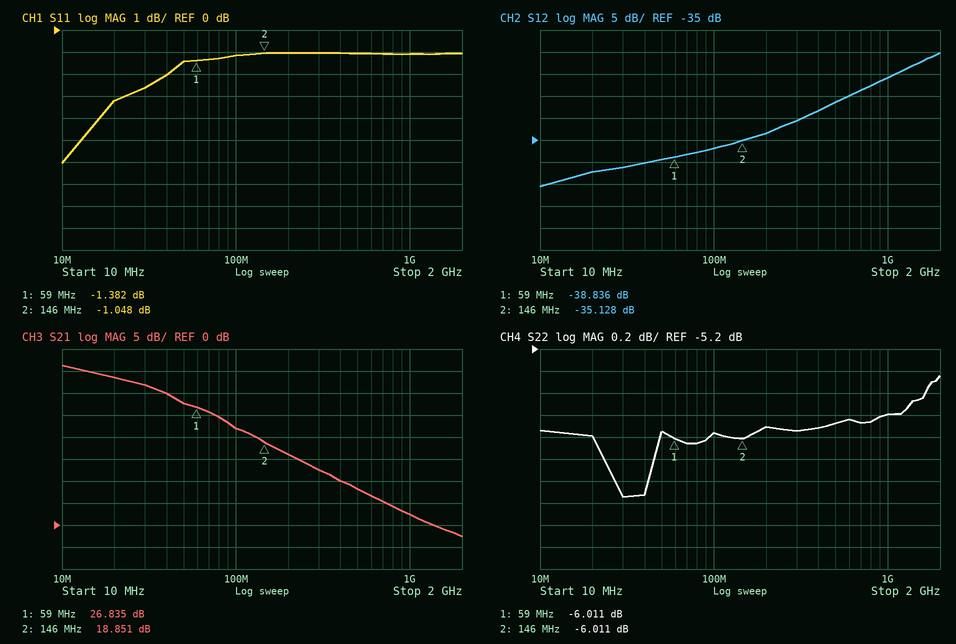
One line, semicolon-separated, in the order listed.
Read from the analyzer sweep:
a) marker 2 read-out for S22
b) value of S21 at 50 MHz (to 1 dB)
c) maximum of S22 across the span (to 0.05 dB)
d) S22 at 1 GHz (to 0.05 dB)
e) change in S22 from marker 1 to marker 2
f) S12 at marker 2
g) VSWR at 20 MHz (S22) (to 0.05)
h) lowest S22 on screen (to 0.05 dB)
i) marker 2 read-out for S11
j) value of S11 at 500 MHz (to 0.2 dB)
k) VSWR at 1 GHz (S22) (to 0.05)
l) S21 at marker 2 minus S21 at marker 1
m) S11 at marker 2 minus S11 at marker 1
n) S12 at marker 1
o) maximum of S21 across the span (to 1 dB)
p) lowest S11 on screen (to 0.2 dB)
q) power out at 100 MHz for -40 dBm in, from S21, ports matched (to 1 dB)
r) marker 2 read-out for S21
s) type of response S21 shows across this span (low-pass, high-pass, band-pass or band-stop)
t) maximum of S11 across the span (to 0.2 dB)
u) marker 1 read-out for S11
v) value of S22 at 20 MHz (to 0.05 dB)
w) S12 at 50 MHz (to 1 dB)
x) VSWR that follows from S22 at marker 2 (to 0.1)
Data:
-6.011 dB; 28 dB; -5.45 dB; -5.80 dB; 0.000 dB; -35.128 dB; 3.00; -6.55 dB; -1.048 dB; -1.0 dB; 3.10; -7.984 dB; 0.334 dB; -38.836 dB; 36 dB; -6.0 dB; -18 dBm; 18.851 dB; low-pass; -1.0 dB; -1.382 dB; -6.00 dB; -39 dB; 3.0
